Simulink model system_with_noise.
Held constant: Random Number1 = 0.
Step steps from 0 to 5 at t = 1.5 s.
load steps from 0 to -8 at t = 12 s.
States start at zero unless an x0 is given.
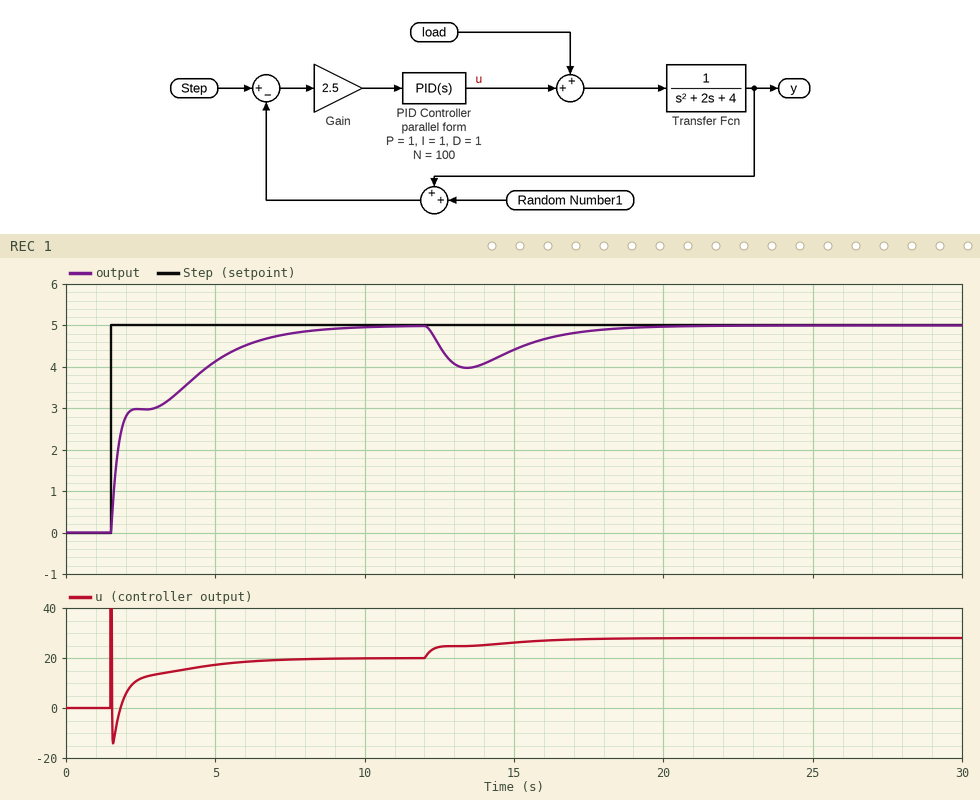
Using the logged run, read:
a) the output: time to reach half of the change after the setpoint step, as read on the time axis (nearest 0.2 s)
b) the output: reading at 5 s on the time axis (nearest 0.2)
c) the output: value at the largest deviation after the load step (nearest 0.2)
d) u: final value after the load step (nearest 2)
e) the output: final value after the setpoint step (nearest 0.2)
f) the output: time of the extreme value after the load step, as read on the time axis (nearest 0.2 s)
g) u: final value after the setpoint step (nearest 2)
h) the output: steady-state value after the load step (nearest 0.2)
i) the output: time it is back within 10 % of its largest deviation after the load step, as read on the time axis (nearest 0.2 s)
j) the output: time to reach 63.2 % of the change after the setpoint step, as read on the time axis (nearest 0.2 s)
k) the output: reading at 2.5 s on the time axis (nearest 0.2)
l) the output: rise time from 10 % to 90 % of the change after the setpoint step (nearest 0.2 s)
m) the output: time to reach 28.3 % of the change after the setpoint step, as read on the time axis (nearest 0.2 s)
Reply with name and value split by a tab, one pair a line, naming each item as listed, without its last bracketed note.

the output: time to reach half of the change after the setpoint step, as read on the time axis	1.8 s
the output: reading at 5 s on the time axis	4.2
the output: value at the largest deviation after the load step	4.0
u: final value after the load step	28
the output: final value after the setpoint step	5.0
the output: time of the extreme value after the load step, as read on the time axis	13.4 s
u: final value after the setpoint step	20
the output: steady-state value after the load step	5.0
the output: time it is back within 10 % of its largest deviation after the load step, as read on the time axis	18.0 s
the output: time to reach 63.2 % of the change after the setpoint step, as read on the time axis	3.4 s
the output: reading at 2.5 s on the time axis	3.0
the output: rise time from 10 % to 90 % of the change after the setpoint step	4.4 s
the output: time to reach 28.3 % of the change after the setpoint step, as read on the time axis	1.6 s
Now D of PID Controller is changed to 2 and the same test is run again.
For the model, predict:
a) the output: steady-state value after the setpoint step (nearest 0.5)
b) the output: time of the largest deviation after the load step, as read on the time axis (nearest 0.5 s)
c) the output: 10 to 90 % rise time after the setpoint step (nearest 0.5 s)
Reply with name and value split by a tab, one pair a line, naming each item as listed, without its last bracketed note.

the output: steady-state value after the setpoint step	5.0
the output: time of the largest deviation after the load step, as read on the time axis	14.0 s
the output: 10 to 90 % rise time after the setpoint step	5.0 s
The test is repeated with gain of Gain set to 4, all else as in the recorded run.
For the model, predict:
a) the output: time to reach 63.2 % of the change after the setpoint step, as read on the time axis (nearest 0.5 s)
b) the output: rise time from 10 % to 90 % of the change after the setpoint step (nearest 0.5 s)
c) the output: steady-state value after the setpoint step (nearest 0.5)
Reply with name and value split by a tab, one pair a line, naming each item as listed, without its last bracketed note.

the output: time to reach 63.2 % of the change after the setpoint step, as read on the time axis	2.0 s
the output: rise time from 10 % to 90 % of the change after the setpoint step	3.5 s
the output: steady-state value after the setpoint step	5.0
